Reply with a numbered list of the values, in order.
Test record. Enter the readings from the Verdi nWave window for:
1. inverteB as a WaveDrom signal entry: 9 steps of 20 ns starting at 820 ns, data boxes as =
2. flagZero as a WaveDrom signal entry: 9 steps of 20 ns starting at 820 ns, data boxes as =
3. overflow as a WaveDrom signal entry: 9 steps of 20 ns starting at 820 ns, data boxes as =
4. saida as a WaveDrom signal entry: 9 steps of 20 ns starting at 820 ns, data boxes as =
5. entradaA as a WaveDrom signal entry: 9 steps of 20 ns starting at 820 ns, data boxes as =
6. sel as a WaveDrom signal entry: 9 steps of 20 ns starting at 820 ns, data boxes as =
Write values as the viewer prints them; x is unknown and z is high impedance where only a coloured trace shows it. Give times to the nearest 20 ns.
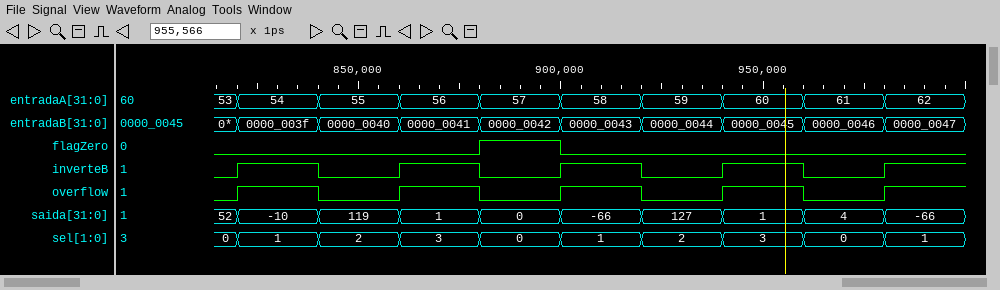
1. {name: 'inverteB', wave: '101010101'}
2. {name: 'flagZero', wave: '0..10....'}
3. {name: 'overflow', wave: '101010101'}
4. {name: 'saida', wave: '=========', data: '-10 119 1 0 -66 127 1 4 -66'}
5. {name: 'entradaA', wave: '=========', data: '54 55 56 57 58 59 60 61 62'}
6. {name: 'sel', wave: '=========', data: '1 2 3 0 1 2 3 0 1'}
